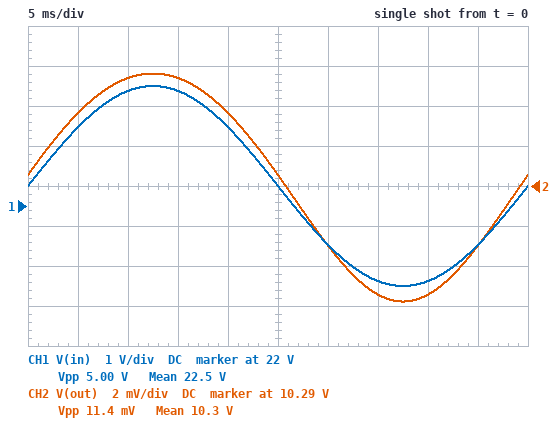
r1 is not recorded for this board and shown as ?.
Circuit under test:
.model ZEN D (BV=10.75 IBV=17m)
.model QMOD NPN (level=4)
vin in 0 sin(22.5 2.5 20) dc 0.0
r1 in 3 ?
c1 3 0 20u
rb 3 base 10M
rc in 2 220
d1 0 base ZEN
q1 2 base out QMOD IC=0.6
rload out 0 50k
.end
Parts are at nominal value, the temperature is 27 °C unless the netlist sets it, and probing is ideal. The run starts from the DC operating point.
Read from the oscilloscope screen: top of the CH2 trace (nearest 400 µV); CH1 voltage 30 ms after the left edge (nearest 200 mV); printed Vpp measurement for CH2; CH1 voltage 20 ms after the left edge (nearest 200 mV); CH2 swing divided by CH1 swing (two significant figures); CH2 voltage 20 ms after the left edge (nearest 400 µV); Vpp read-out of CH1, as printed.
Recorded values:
10.2996 V
21.0 V
11.4 mV
24.0 V
0.0023
10.2976 V
5.00 V
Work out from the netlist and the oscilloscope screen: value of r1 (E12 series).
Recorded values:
4.7 mΩ
